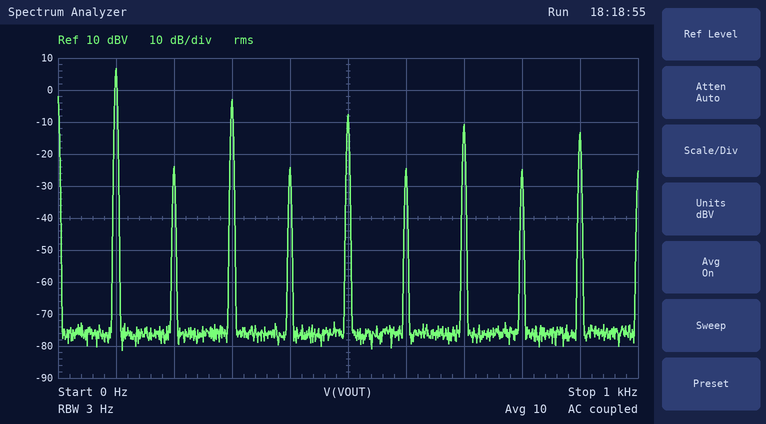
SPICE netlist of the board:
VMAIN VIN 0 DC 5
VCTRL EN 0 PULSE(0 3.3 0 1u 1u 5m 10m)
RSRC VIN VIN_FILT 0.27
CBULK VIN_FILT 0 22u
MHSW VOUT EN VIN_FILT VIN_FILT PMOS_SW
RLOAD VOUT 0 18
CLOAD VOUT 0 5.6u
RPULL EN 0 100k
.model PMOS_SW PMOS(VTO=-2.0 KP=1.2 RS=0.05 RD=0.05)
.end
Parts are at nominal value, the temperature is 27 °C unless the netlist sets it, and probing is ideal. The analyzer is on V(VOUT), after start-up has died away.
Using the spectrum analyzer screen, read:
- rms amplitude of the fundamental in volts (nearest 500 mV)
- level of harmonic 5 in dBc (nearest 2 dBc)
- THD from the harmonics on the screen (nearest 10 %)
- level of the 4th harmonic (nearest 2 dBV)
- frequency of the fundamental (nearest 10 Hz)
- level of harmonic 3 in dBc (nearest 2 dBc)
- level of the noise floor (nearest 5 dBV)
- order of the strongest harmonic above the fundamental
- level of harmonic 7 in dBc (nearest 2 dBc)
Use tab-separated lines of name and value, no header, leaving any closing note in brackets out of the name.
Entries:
rms amplitude of the fundamental in volts	2.0 V
level of harmonic 5 in dBc	-14 dBc
THD from the harmonics on the screen	40 %
level of the 4th harmonic	-24 dBV
frequency of the fundamental	100 Hz
level of harmonic 3 in dBc	-10 dBc
level of the noise floor	-75 dBV
order of the strongest harmonic above the fundamental	3
level of harmonic 7 in dBc	-18 dBc
